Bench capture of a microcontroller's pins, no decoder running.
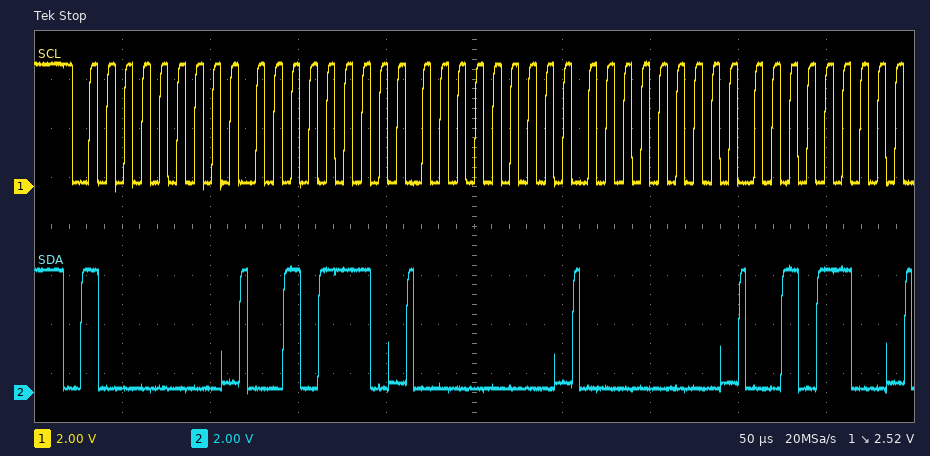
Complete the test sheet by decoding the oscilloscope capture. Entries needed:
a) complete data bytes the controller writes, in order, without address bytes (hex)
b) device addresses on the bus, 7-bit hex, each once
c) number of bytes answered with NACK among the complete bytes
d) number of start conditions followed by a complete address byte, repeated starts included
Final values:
2E 00 00 2C
0x40
0
1
